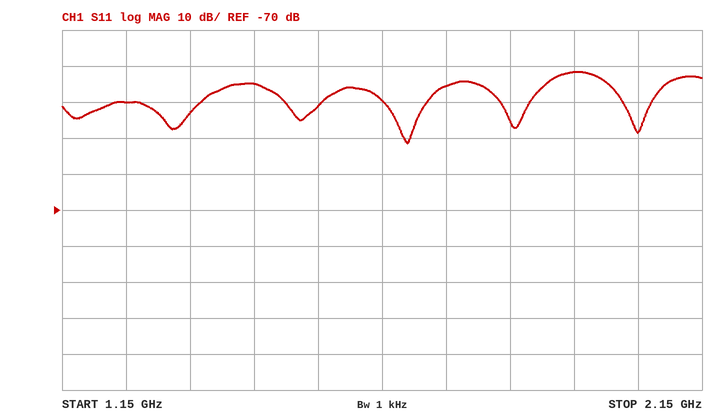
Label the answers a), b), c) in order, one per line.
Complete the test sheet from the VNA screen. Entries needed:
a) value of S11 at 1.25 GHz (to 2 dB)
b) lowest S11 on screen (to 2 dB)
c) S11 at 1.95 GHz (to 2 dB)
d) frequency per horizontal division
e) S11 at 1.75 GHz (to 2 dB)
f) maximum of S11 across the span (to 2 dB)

a) -40 dB
b) -52 dB
c) -32 dB
d) 100 MHz
e) -36 dB
f) -32 dB
